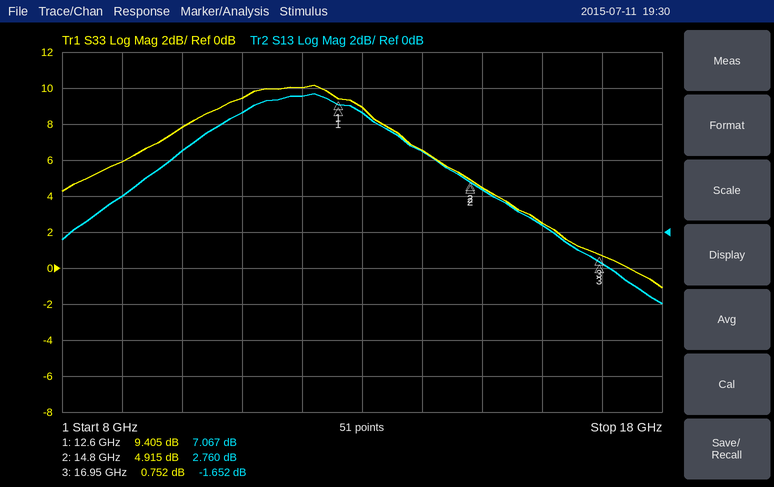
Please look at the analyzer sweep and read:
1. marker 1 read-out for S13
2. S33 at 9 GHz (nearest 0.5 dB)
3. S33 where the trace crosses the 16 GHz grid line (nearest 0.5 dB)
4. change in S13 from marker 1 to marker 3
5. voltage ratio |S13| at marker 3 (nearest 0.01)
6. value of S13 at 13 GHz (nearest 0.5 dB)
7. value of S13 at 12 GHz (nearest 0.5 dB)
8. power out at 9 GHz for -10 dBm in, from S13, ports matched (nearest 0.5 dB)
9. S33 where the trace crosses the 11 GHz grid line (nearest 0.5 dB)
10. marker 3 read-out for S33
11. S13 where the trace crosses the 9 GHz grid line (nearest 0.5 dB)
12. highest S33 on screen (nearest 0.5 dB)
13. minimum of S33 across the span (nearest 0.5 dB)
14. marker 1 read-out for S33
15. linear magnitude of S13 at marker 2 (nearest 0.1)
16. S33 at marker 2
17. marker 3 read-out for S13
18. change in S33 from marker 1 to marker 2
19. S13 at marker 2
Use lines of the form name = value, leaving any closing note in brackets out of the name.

marker 1 read-out for S13 = 7.067 dB
S33 at 9 GHz = 6.0 dB
S33 where the trace crosses the 16 GHz grid line = 2.5 dB
change in S13 from marker 1 to marker 3 = -8.719 dB
voltage ratio |S13| at marker 3 = 0.83
value of S13 at 13 GHz = 6.5 dB
value of S13 at 12 GHz = 7.5 dB
power out at 9 GHz for -10 dBm in, from S13, ports matched = -8.0 dBm
S33 where the trace crosses the 11 GHz grid line = 9.5 dB
marker 3 read-out for S33 = 0.752 dB
S13 where the trace crosses the 9 GHz grid line = 2.0 dB
highest S33 on screen = 10.0 dB
minimum of S33 across the span = -1.0 dB
marker 1 read-out for S33 = 9.405 dB
linear magnitude of S13 at marker 2 = 1.4
S33 at marker 2 = 4.915 dB
marker 3 read-out for S13 = -1.652 dB
change in S33 from marker 1 to marker 2 = -4.490 dB
S13 at marker 2 = 2.760 dB
